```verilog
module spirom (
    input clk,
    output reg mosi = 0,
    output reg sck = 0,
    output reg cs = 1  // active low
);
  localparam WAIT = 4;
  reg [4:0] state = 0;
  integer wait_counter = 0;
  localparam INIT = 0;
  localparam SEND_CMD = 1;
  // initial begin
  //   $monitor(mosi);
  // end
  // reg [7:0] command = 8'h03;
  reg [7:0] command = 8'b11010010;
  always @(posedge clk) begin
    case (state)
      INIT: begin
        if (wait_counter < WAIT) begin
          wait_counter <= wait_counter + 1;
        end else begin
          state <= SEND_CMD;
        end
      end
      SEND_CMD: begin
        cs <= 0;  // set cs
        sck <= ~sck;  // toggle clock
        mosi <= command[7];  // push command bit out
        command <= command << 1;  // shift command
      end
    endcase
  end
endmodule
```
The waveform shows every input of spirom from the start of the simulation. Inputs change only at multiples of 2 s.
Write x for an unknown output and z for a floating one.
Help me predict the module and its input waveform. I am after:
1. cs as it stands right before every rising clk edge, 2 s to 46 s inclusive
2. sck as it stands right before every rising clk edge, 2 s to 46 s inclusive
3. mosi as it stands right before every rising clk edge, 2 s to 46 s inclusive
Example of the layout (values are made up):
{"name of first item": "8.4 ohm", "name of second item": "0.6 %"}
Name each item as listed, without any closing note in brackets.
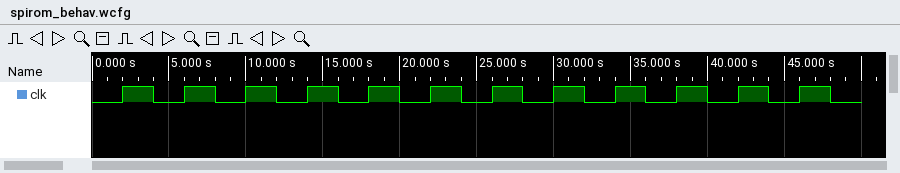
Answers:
{"cs as it stands right before every rising clk edge, 2 s to 46 s inclusive": "1 1 1 1 1 1 0 0 0 0 0 0", "sck as it stands right before every rising clk edge, 2 s to 46 s inclusive": "0 0 0 0 0 0 1 0 1 0 1 0", "mosi as it stands right before every rising clk edge, 2 s to 46 s inclusive": "0 0 0 0 0 0 1 1 0 1 0 0"}
